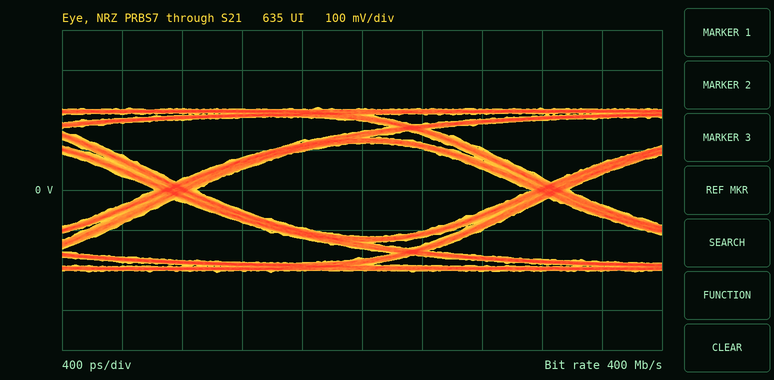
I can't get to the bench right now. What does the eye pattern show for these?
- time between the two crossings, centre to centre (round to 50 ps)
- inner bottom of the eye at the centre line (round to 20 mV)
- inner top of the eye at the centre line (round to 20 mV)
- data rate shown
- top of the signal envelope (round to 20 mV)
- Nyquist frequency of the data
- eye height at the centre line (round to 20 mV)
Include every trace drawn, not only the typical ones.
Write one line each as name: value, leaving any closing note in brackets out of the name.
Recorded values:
time between the two crossings, centre to centre: 2.50 ns
inner bottom of the eye at the centre line: -120 mV
inner top of the eye at the centre line: 120 mV
data rate shown: 400 Mb/s
top of the signal envelope: 200 mV
Nyquist frequency of the data: 200 MHz
eye height at the centre line: 240 mV
